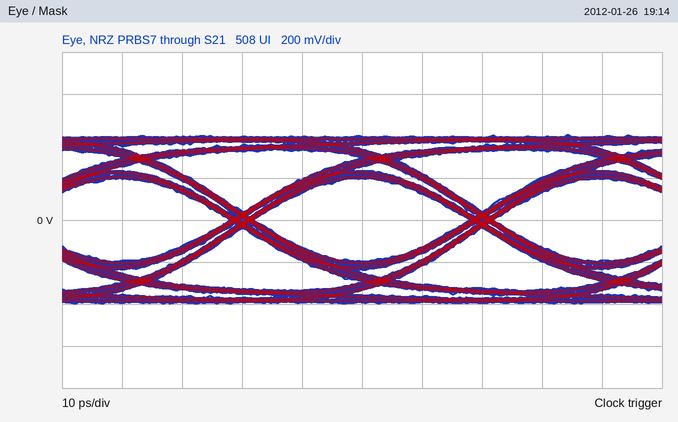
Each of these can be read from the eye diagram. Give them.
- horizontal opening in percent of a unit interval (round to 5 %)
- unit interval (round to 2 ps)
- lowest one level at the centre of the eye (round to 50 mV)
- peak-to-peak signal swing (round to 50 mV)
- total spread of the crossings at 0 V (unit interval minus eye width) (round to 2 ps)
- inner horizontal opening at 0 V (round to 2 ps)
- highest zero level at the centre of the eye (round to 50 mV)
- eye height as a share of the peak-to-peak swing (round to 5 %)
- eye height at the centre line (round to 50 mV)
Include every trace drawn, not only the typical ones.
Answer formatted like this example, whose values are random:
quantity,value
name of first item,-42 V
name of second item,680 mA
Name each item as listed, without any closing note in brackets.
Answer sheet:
quantity,value
horizontal opening in percent of a unit interval,90 %
unit interval,40 ps
lowest one level at the centre of the eye,200 mV
peak-to-peak signal swing,800 mV
total spread of the crossings at 0 V (unit interval minus eye width),4 ps
inner horizontal opening at 0 V,36 ps
highest zero level at the centre of the eye,-200 mV
eye height as a share of the peak-to-peak swing,50 %
eye height at the centre line,400 mV
